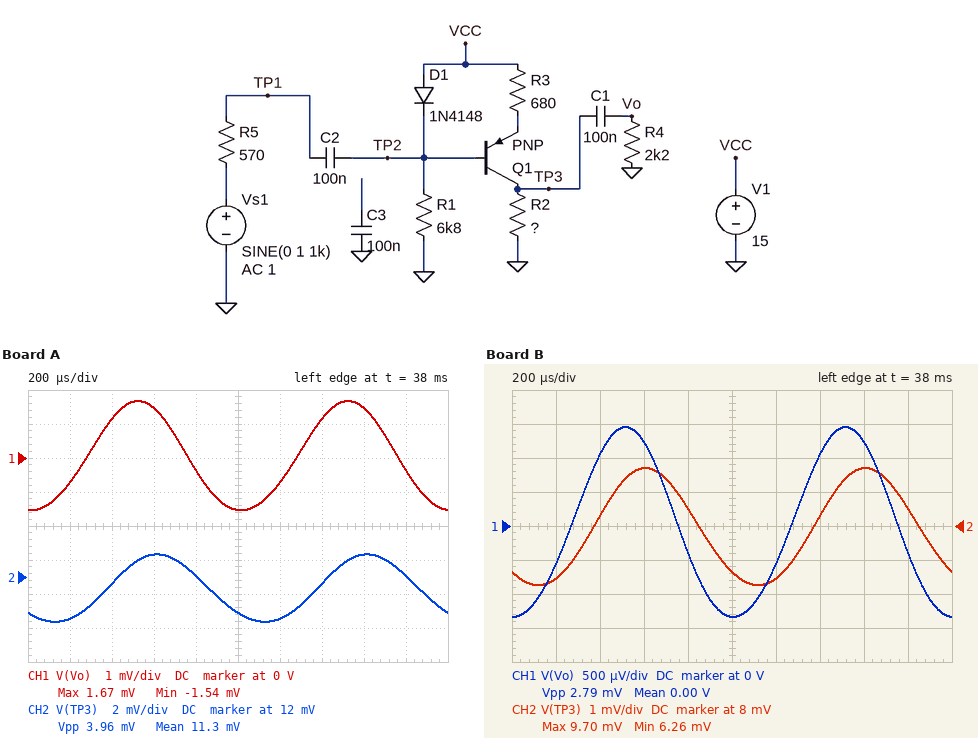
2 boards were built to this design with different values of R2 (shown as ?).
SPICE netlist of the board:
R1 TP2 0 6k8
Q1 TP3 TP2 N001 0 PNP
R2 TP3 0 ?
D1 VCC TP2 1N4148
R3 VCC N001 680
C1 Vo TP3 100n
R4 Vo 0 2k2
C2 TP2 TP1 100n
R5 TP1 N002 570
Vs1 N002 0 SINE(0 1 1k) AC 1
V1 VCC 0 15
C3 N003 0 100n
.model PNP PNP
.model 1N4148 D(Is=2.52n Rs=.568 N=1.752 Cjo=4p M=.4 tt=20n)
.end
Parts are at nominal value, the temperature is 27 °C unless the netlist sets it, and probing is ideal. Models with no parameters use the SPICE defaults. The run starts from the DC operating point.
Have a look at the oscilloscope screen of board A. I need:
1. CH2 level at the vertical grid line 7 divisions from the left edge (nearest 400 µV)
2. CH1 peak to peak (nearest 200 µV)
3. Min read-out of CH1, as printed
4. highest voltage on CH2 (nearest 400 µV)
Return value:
11.6 mV
3.2 mV
-1.54 mV
13.2 mV
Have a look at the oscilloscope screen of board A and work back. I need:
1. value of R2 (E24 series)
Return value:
4.7 kΩ
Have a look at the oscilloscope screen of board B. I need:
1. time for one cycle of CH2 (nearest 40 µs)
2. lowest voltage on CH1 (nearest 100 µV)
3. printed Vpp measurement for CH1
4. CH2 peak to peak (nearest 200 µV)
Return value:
1.00 ms
-1.3 mV
2.79 mV
3.4 mV
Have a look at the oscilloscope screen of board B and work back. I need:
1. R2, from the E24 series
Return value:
3.3 kΩ
